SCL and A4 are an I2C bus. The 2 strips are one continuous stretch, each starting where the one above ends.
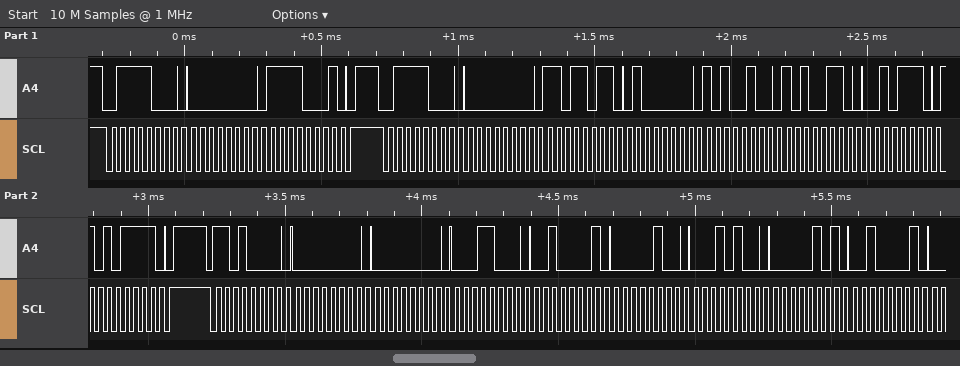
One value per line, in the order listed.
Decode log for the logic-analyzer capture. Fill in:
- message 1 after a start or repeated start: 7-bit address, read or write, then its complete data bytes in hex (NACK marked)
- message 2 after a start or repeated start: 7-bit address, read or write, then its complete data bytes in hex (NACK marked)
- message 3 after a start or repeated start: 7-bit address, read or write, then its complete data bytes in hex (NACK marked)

0x3C write: 00 F1
0x3C write: 00 DB 40 A4 A6 2E AF
0x68 write: 00 00 18 21 04 14 05 21
